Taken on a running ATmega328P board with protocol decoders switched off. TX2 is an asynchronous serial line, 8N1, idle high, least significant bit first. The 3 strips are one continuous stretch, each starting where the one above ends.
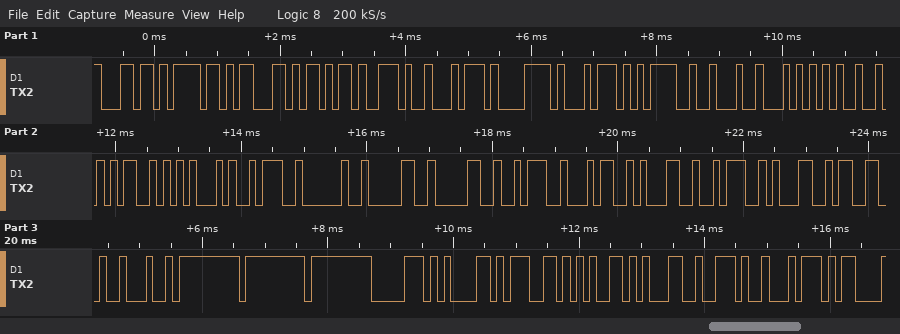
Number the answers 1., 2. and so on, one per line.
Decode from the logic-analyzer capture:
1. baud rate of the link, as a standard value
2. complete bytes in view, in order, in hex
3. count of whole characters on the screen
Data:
1. 9600 baud
2. 6C 6F 63 6B 2E 74 78 74 3D 22 54 49 4D 45 3A 20 30 30 3A 34 31 3A 31 33 22 FF FF FF 70 61 67 65 31 2E 74
3. 35
